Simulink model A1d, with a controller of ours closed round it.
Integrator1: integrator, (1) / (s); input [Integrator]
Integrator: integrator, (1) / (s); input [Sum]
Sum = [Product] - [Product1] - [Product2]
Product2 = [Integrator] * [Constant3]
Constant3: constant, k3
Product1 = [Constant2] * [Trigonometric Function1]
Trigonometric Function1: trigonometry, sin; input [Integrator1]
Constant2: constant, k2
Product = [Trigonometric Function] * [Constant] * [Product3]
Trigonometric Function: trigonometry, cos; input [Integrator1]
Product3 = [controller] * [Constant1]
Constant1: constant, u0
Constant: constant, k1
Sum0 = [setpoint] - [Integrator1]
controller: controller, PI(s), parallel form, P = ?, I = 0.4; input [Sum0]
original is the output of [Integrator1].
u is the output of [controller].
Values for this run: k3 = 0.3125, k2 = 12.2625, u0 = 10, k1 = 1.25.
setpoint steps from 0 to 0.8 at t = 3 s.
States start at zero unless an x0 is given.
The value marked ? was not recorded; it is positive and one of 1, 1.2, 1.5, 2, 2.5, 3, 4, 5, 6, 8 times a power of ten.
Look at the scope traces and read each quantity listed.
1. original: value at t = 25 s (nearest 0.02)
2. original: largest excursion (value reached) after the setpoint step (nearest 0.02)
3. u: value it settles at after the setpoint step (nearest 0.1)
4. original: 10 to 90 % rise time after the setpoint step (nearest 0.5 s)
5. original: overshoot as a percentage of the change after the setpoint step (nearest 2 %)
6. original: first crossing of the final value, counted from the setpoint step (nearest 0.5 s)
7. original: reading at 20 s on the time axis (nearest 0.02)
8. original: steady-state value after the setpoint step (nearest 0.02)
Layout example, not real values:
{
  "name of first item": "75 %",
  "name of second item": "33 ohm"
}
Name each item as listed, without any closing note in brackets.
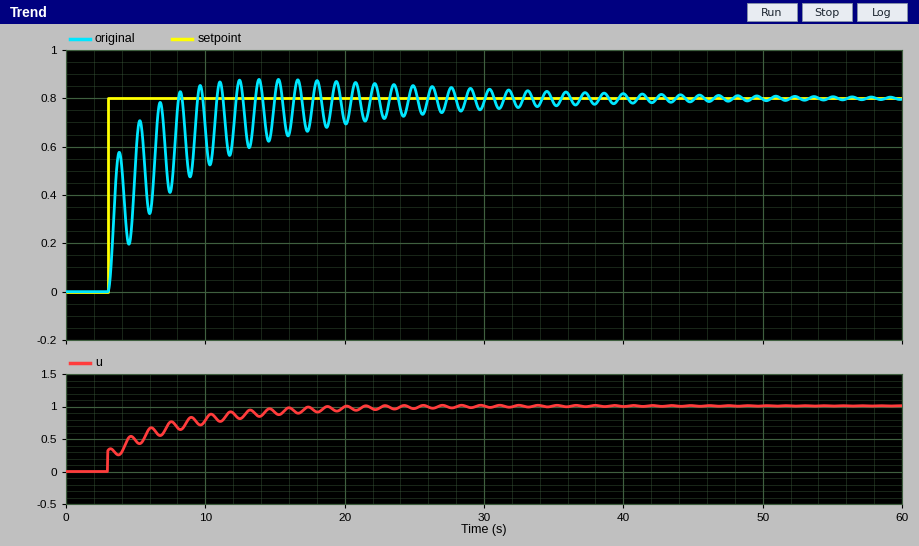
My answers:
{
  "original: value at t = 25 s": "0.84",
  "original: largest excursion (value reached) after the setpoint step": "0.88",
  "u: value it settles at after the setpoint step": "1.0",
  "original: 10 to 90 % rise time after the setpoint step": "3.5 s",
  "original: overshoot as a percentage of the change after the setpoint step": "10 %",
  "original: first crossing of the final value, counted from the setpoint step": "5.0 s",
  "original: reading at 20 s on the time axis": "0.70",
  "original: steady-state value after the setpoint step": "0.80"
}
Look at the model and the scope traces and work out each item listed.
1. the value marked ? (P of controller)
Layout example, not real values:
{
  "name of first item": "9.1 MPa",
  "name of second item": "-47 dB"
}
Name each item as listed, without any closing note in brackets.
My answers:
{
  "the value marked ?": "0.4"
}
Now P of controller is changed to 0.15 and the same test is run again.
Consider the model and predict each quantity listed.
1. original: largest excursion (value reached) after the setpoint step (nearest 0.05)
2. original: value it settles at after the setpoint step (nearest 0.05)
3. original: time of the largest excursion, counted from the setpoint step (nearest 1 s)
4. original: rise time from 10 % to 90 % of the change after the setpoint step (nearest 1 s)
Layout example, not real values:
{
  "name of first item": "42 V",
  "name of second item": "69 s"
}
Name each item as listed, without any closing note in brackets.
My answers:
{
  "original: largest excursion (value reached) after the setpoint step": "0.85",
  "original: value it settles at after the setpoint step": "0.80",
  "original: time of the largest excursion, counted from the setpoint step": "15 s",
  "original: rise time from 10 % to 90 % of the change after the setpoint step": "4 s"
}
